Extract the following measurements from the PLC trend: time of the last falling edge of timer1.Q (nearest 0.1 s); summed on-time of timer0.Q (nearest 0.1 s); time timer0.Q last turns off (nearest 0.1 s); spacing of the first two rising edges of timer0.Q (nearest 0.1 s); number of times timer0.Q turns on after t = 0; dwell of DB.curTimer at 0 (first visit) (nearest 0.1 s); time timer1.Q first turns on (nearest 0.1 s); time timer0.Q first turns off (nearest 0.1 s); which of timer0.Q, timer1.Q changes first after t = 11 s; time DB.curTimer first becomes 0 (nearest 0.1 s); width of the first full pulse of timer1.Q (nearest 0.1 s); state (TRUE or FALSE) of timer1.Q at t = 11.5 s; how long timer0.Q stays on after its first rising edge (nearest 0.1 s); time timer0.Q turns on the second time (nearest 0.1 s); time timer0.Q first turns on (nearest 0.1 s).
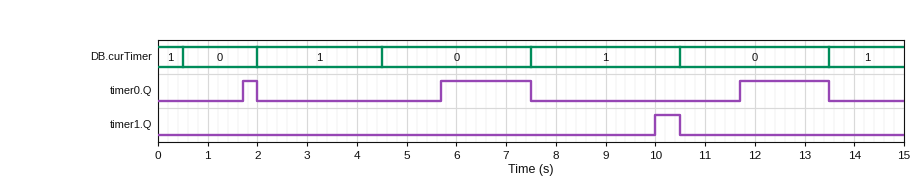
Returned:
10.5 s
3.9 s
13.5 s
4.0 s
3
1.5 s
10.0 s
2.0 s
timer0.Q
0.5 s
0.5 s
FALSE
0.3 s
5.7 s
1.7 s
